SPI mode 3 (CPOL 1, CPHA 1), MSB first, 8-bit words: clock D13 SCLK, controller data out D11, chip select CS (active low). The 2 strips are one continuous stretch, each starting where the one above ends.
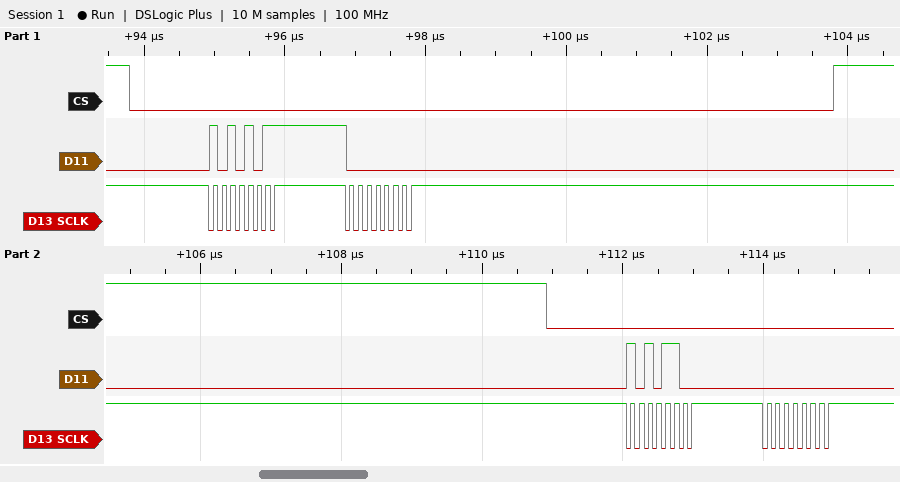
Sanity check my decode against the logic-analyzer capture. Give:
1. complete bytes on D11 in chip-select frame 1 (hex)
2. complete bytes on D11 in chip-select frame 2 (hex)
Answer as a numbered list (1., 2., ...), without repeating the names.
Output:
1. AB 00
2. AC 00
